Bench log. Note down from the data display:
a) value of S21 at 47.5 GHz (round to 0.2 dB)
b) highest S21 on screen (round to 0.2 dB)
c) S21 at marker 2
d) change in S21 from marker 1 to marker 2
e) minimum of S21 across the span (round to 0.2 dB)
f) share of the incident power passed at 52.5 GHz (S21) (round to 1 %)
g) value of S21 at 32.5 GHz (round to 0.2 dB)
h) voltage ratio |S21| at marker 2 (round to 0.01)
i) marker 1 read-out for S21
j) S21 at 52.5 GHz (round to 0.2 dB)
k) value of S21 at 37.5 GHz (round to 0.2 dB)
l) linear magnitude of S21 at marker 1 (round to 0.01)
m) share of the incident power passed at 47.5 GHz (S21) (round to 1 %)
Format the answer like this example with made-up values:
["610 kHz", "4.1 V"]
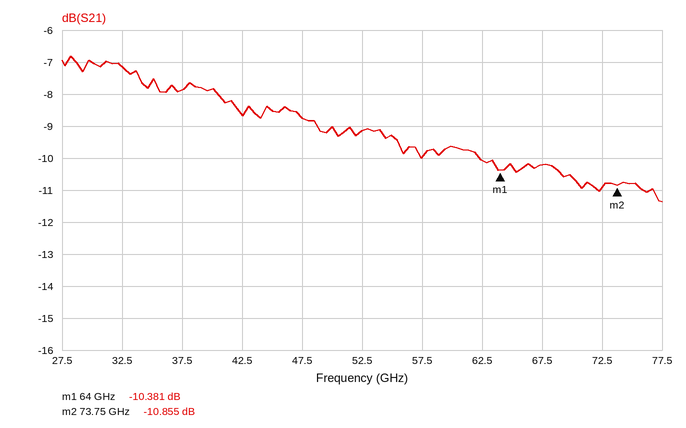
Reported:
["-8.8 dB", "-6.8 dB", "-10.855 dB", "-0.474 dB", "-11.4 dB", "12 %", "-7.2 dB", "0.29", "-10.381 dB", "-9.2 dB", "-7.8 dB", "0.30", "13 %"]
